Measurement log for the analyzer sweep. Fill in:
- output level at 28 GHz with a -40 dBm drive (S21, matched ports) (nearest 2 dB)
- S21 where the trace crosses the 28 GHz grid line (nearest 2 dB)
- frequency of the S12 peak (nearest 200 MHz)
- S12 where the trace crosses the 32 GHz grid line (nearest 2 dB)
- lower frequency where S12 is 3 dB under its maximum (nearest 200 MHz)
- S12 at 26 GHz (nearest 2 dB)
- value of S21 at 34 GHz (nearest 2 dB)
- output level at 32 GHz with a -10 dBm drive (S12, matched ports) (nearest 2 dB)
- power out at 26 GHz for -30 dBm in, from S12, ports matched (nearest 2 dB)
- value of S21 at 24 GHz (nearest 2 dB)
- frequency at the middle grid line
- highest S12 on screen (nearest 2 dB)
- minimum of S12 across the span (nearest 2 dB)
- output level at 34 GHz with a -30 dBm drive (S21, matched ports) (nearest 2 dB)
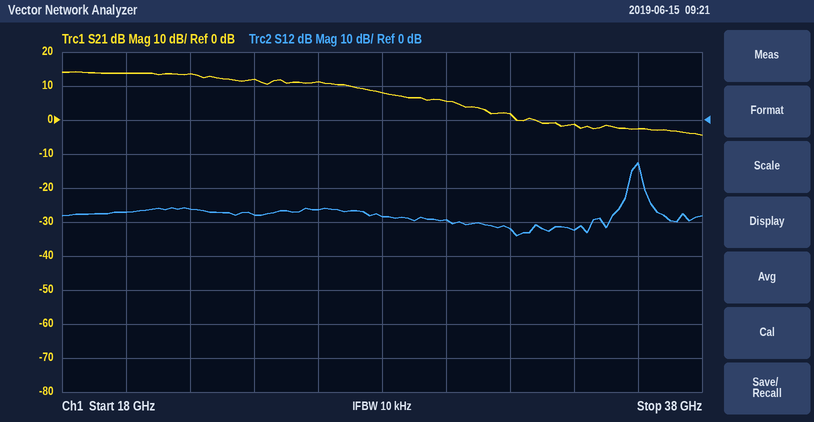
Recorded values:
-32 dBm
8 dB
36.0 GHz
-32 dB
35.8 GHz
-26 dB
-2 dB
-42 dBm
-56 dBm
12 dB
28 GHz
-12 dB
-34 dB
-32 dBm
